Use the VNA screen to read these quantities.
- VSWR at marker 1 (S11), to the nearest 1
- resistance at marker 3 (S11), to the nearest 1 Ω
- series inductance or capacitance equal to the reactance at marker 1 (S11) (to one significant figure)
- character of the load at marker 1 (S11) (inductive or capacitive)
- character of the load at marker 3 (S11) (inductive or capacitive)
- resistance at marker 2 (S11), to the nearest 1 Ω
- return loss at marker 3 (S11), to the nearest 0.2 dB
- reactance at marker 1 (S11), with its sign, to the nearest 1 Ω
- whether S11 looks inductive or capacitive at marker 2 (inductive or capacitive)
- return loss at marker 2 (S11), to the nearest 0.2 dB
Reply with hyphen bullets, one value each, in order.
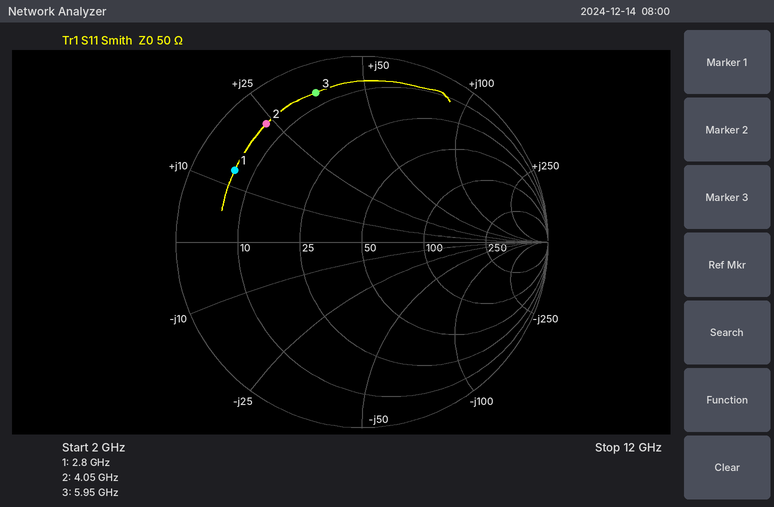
- 8
- 7 Ω
- 700 pH
- inductive
- inductive
- 6 Ω
- 1.6 dB
- +13 Ω
- inductive
- 1.8 dB
